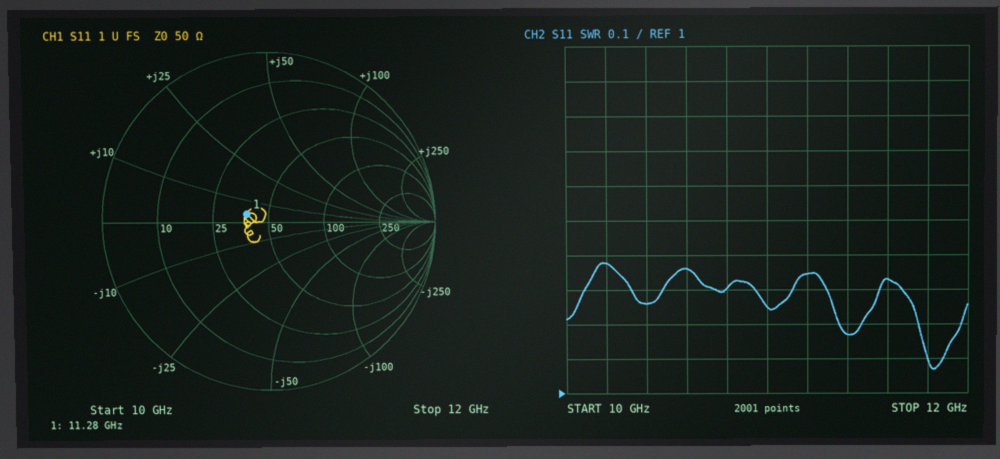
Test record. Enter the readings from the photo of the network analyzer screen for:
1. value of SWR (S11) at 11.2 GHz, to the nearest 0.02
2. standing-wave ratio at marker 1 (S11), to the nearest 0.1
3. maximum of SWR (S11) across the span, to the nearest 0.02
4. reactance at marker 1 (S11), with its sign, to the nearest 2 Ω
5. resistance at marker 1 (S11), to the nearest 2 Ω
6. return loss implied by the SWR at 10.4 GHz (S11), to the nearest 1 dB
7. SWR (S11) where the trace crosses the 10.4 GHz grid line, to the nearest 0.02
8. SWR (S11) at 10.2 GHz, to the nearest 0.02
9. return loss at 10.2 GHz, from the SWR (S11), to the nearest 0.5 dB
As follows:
1.34
1.3
1.38
+4 Ω
38 Ω
19 dB
1.26
1.38
16.0 dB
